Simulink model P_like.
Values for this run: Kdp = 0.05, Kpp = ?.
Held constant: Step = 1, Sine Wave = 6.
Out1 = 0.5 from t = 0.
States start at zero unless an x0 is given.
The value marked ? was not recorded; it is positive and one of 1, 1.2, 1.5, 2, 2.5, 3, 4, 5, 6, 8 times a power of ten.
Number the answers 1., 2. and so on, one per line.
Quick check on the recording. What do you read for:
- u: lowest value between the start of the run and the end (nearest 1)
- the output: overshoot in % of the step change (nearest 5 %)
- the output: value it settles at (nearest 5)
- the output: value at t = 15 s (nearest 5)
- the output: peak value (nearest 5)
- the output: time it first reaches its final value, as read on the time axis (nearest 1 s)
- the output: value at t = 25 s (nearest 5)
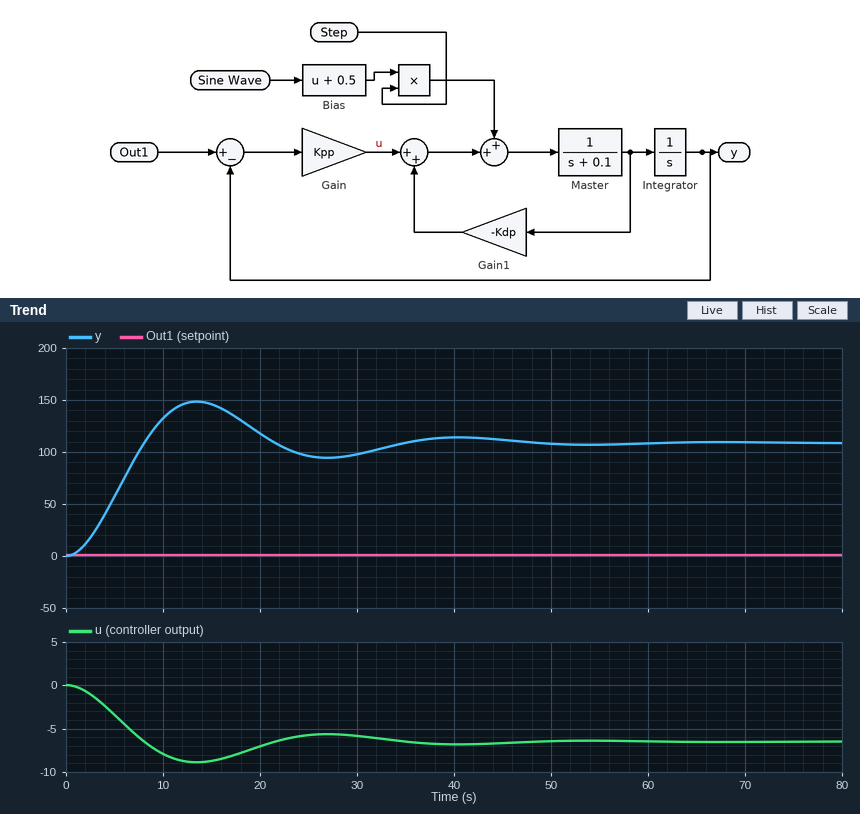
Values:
1. -9
2. 35 %
3. 110
4. 145
5. 150
6. 8 s
7. 95
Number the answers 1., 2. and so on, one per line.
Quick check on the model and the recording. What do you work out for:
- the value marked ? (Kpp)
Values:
1. 0.06
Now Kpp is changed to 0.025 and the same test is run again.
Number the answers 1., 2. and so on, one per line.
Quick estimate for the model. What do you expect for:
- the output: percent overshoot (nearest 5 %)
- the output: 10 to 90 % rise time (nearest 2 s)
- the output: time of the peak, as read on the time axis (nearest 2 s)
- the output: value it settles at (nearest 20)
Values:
1. 20 %
2. 10 s
3. 22 s
4. 260
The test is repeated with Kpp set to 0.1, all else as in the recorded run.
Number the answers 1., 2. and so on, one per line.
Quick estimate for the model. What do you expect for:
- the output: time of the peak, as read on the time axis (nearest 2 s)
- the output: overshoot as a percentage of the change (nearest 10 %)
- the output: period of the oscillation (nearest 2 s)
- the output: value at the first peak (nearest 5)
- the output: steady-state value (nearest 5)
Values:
1. 10 s
2. 50 %
3. 20 s
4. 95
5. 65
